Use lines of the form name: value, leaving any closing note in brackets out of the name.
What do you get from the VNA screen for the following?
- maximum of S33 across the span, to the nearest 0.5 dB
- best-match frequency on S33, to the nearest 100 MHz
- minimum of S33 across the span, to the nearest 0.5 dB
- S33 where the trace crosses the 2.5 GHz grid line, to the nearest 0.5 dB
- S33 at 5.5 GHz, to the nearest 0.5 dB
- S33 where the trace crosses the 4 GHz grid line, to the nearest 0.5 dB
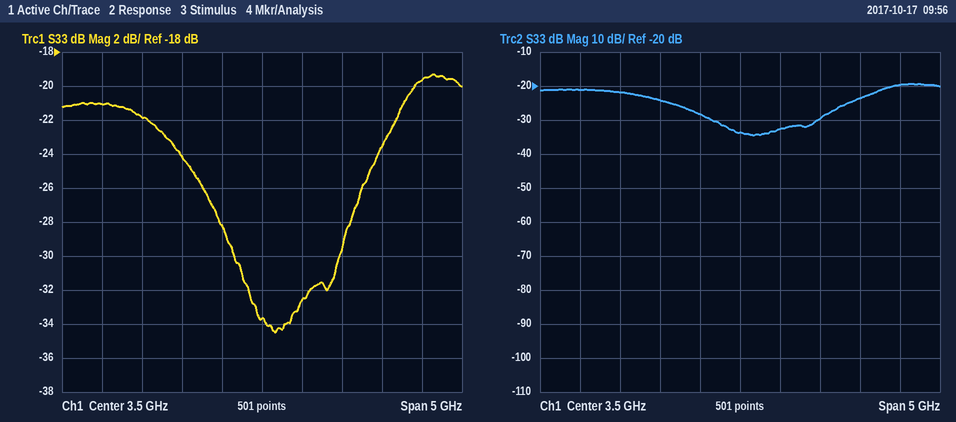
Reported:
maximum of S33 across the span, to the nearest 0.5 dB: -19.5 dB
best-match frequency on S33, to the nearest 100 MHz: 3.7 GHz
minimum of S33 across the span, to the nearest 0.5 dB: -34.5 dB
S33 where the trace crosses the 2.5 GHz grid line, to the nearest 0.5 dB: -24.0 dB
S33 at 5.5 GHz, to the nearest 0.5 dB: -19.5 dB
S33 where the trace crosses the 4 GHz grid line, to the nearest 0.5 dB: -32.5 dB
